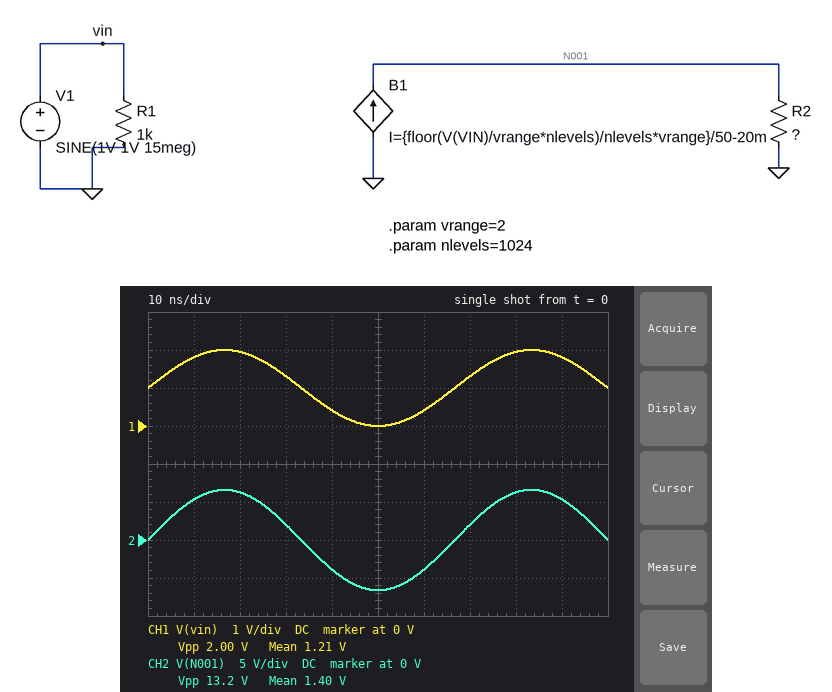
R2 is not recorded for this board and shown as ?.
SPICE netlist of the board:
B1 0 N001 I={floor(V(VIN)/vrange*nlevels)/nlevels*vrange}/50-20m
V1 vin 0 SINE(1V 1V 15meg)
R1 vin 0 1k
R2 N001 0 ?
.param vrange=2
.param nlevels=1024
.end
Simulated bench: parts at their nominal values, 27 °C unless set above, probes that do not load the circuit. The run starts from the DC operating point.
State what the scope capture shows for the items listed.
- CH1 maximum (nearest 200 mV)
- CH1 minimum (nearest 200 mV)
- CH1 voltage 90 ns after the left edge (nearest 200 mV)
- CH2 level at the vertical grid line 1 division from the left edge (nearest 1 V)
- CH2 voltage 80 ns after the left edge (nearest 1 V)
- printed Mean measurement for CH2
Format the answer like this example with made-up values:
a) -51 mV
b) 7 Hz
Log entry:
a) 2.0 V
b) 0 V
c) 1.8 V
d) 5 V
e) 6 V
f) 1.40 V
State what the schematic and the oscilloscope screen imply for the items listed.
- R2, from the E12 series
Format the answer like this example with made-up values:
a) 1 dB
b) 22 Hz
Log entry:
a) 330 Ω
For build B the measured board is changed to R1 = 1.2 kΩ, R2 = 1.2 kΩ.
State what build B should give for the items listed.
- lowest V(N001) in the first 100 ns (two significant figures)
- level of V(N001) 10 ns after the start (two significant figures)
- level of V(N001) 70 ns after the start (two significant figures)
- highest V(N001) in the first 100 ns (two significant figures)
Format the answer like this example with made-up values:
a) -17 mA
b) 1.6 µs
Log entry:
a) -24 V
b) 19 V
c) 7.4 V
d) 24 V
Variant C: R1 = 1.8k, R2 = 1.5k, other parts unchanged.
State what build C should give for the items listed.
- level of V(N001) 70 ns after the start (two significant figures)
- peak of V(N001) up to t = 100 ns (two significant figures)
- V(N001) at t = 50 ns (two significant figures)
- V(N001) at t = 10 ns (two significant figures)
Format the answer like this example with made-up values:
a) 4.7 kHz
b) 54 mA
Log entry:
a) 9.2 V
b) 30 V
c) -30 V
d) 24 V
